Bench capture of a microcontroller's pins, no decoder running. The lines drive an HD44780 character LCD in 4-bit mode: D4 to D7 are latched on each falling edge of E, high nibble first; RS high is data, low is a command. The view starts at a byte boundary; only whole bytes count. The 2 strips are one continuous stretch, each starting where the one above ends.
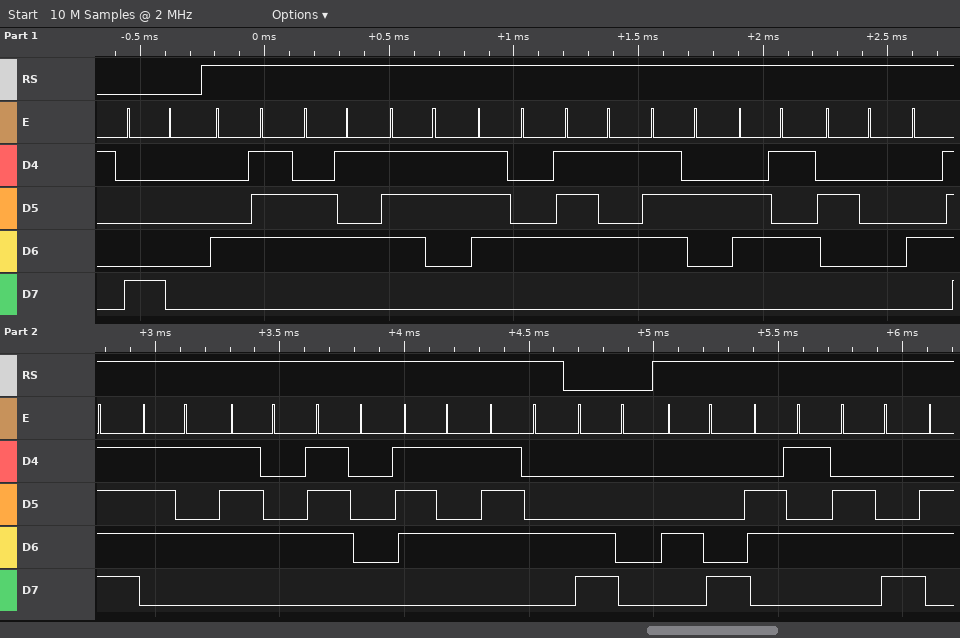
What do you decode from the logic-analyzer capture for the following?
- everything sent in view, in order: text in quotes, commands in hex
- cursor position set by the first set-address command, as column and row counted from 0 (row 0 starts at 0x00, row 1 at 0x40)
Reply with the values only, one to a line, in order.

0x80 "Gesture Output" 0xC0 "Hel"
column 0, row 0
